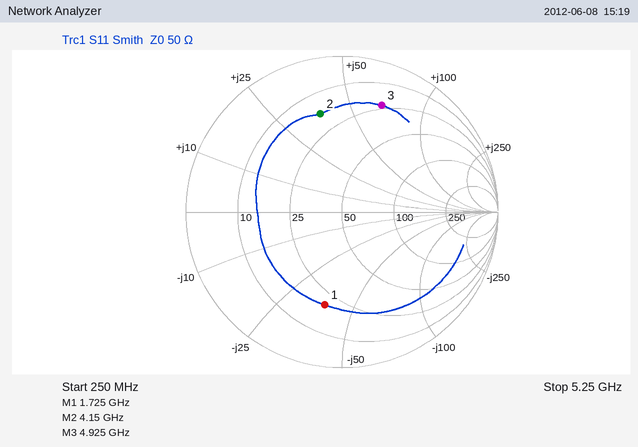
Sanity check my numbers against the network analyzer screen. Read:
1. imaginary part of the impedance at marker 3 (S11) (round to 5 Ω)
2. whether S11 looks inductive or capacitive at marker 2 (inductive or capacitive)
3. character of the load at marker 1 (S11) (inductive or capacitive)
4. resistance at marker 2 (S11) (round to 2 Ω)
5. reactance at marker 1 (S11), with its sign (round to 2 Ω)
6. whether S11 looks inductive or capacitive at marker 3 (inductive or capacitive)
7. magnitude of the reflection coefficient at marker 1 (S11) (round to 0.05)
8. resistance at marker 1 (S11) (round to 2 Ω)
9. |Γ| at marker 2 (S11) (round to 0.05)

+65 Ω
inductive
capacitive
18 Ω
-38 Ω
inductive
0.60
20 Ω
0.65
